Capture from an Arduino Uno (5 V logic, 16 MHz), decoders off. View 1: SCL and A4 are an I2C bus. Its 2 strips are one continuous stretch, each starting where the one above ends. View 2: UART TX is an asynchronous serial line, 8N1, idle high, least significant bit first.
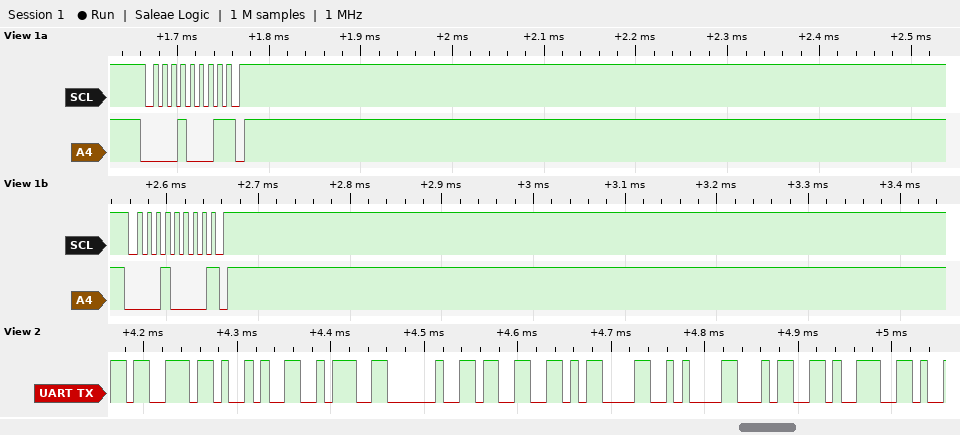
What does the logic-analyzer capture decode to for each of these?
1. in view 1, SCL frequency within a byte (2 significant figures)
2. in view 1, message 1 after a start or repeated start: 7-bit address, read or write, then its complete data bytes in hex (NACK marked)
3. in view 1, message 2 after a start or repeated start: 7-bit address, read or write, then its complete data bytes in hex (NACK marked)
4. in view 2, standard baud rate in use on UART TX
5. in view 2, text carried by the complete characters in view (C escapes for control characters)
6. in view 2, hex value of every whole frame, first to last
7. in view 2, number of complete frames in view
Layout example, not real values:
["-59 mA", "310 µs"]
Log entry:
["100 kHz", "0x08 read NACK", "0x08 write NACK", "115200 baud", "\"s): 3\\r\\n49\"", "73 29 3A 20 33 0D 0A 34 39", "9"]
